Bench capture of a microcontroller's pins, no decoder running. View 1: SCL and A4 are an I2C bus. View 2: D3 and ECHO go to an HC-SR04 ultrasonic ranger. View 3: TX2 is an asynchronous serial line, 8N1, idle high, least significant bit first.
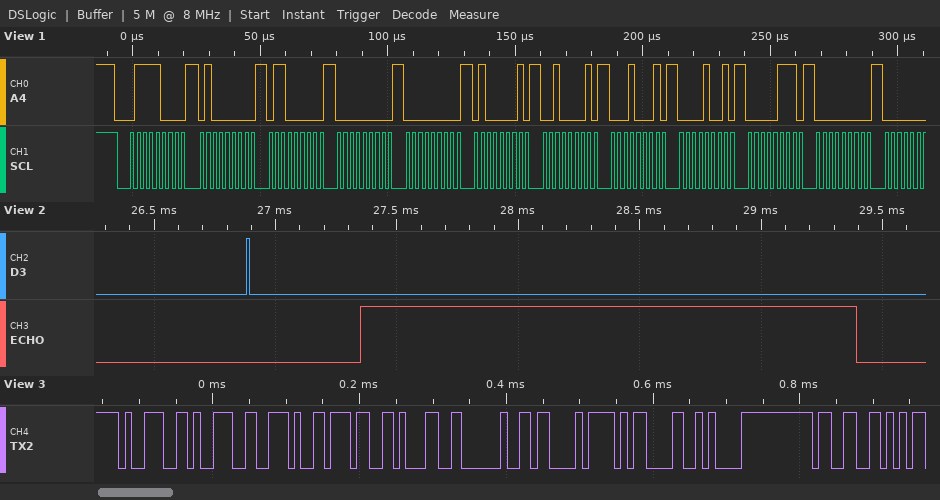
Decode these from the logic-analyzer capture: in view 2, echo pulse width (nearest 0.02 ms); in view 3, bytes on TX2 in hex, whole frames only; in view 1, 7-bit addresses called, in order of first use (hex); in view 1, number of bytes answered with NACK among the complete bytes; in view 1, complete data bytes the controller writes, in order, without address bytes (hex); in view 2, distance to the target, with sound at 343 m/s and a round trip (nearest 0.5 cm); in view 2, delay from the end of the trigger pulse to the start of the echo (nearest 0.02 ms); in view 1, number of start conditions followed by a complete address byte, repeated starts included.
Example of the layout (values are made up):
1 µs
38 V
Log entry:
2.04 ms
39 39 2E 37 31 20 43 0D 0A 33
0x3C
0
40 60 00 00 41 21 11 09 07 00
35 cm
0.46 ms
1
